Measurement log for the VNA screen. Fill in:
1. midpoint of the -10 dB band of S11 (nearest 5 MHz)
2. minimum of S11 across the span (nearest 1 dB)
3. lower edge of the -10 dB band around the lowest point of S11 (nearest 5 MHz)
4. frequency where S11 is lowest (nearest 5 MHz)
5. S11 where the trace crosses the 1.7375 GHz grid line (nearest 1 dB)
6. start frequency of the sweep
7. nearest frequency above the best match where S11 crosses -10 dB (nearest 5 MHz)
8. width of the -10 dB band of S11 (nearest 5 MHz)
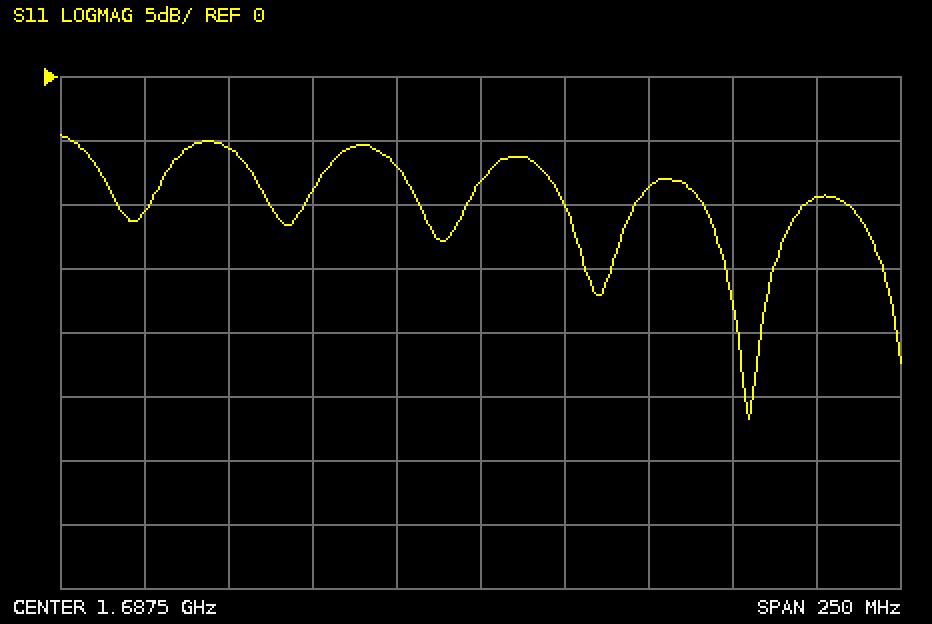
1.770 GHz
-27 dB
1.755 GHz
1.765 GHz
-9 dB
1.5625 GHz
1.785 GHz
30 MHz
